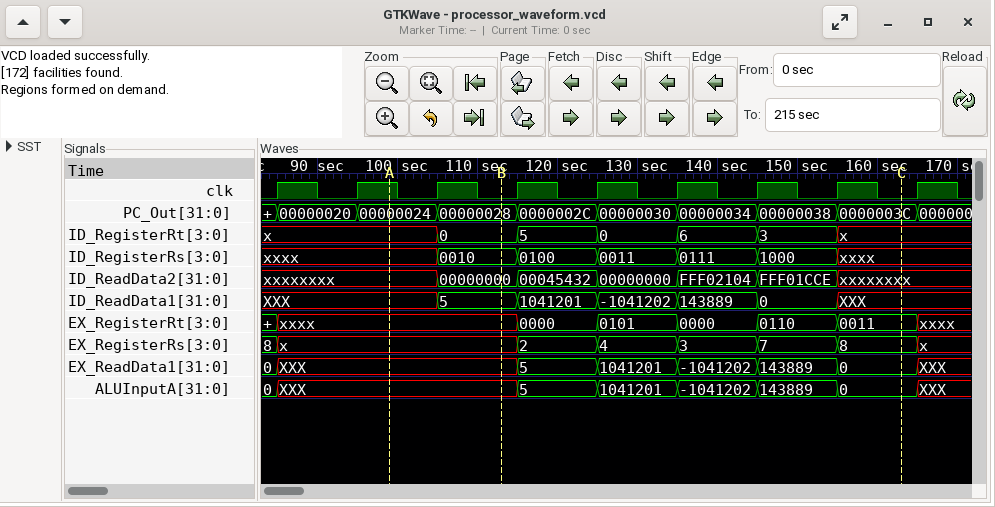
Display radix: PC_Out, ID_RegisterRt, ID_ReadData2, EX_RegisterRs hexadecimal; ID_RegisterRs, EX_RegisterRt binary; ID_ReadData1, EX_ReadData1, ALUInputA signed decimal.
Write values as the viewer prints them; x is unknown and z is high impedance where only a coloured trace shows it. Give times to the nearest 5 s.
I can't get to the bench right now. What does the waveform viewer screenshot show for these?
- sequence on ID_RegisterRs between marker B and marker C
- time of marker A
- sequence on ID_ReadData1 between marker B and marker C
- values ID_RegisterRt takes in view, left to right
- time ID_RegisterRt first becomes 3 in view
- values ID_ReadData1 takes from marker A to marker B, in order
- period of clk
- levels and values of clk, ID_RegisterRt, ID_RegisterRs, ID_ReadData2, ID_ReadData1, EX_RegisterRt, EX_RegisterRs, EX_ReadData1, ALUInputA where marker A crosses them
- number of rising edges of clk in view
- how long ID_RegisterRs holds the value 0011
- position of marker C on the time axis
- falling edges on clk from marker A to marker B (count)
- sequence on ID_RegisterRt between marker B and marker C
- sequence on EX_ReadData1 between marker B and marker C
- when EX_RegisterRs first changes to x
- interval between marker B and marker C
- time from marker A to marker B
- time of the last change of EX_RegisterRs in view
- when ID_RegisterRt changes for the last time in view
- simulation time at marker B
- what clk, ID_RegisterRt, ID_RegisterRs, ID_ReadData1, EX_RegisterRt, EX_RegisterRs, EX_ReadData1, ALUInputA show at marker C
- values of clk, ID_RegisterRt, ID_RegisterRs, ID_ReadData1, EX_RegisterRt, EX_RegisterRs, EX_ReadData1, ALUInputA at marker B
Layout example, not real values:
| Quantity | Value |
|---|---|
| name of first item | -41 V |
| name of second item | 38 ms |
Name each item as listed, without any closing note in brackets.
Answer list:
| Quantity | Value |
|---|---|
| sequence on ID_RegisterRs between marker B and marker C | 0010, 0100, 0011, 0111, 1000, xxxx |
| time of marker A | 100 s |
| sequence on ID_ReadData1 between marker B and marker C | 5, 1041201, -1041202, 143889, 0, XXX |
| values ID_RegisterRt takes in view, left to right | x, 0, 5, 0, 6, 3, x |
| time ID_RegisterRt first becomes 3 in view | 145 s |
| values ID_ReadData1 takes from marker A to marker B, in order | XXX, 5 |
| period of clk | 10 s |
| levels and values of clk, ID_RegisterRt, ID_RegisterRs, ID_ReadData2, ID_ReadData1, EX_RegisterRt, EX_RegisterRs, EX_ReadData1, ALUInputA where marker A crosses them | clk=1, ID_RegisterRt=x, ID_RegisterRs=xxxx, ID_ReadData2=xxxxxxxx, ID_ReadData1=XXX, EX_RegisterRt=xxxx, EX_RegisterRs=x, EX_ReadData1=XXX, ALUInputA=XXX |
| number of rising edges of clk in view | 9 |
| how long ID_RegisterRs holds the value 0011 | 10 s |
| position of marker C on the time axis | 165 s |
| falling edges on clk from marker A to marker B | 2 |
| sequence on ID_RegisterRt between marker B and marker C | 0, 5, 0, 6, 3, x |
| sequence on EX_ReadData1 between marker B and marker C | XXX, 5, 1041201, -1041202, 143889, 0 |
| when EX_RegisterRs first changes to x | 85 s |
| interval between marker B and marker C | 50 s |
| time from marker A to marker B | 15 s |
| time of the last change of EX_RegisterRs in view | 165 s |
| when ID_RegisterRt changes for the last time in view | 155 s |
| simulation time at marker B | 115 s |
| what clk, ID_RegisterRt, ID_RegisterRs, ID_ReadData1, EX_RegisterRt, EX_RegisterRs, EX_ReadData1, ALUInputA show at marker C | clk=0, ID_RegisterRt=x, ID_RegisterRs=xxxx, ID_ReadData1=XXX, EX_RegisterRt=0011, EX_RegisterRs=8, EX_ReadData1=0, ALUInputA=0 |
| values of clk, ID_RegisterRt, ID_RegisterRs, ID_ReadData1, EX_RegisterRt, EX_RegisterRs, EX_ReadData1, ALUInputA at marker B | clk=0, ID_RegisterRt=0, ID_RegisterRs=0010, ID_ReadData1=5, EX_RegisterRt=xxxx, EX_RegisterRs=x, EX_ReadData1=XXX, ALUInputA=XXX |
